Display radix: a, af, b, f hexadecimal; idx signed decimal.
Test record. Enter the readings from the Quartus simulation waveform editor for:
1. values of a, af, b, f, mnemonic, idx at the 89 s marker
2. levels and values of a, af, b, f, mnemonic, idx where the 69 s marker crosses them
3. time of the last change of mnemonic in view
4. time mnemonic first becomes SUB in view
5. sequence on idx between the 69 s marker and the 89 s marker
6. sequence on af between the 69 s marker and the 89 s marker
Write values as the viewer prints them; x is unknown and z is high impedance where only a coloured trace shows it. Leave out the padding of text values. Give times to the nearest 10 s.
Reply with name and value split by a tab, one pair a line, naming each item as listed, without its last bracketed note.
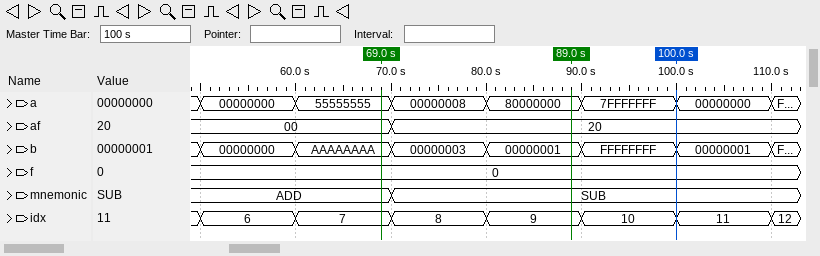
values of a, af, b, f, mnemonic, idx at the 89 s marker	a=80000000, af=20, b=00000001, f=0, mnemonic=SUB, idx=9
levels and values of a, af, b, f, mnemonic, idx where the 69 s marker crosses them	a=55555555, af=00, b=AAAAAAAA, f=0, mnemonic=ADD, idx=7
time of the last change of mnemonic in view	70 s
time mnemonic first becomes SUB in view	70 s
sequence on idx between the 69 s marker and the 89 s marker	7, 8, 9
sequence on af between the 69 s marker and the 89 s marker	00, 20
